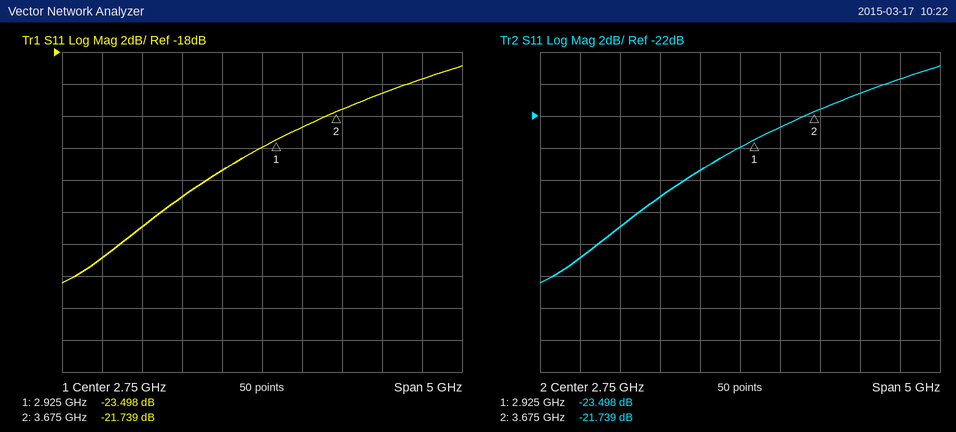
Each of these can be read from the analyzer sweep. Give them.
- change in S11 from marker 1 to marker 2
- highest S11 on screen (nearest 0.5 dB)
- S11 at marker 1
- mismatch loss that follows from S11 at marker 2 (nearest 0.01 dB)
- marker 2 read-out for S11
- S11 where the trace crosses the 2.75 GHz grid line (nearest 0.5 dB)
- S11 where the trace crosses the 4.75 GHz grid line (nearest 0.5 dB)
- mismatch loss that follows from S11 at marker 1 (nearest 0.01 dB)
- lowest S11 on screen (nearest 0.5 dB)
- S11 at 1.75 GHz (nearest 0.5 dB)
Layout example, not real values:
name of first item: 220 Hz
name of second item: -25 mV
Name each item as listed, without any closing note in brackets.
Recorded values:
change in S11 from marker 1 to marker 2: 1.759 dB
highest S11 on screen: -19.0 dB
S11 at marker 1: -23.498 dB
mismatch loss that follows from S11 at marker 2: 0.03 dB
marker 2 read-out for S11: -21.739 dB
S11 where the trace crosses the 2.75 GHz grid line: -24.0 dB
S11 where the trace crosses the 4.75 GHz grid line: -19.5 dB
mismatch loss that follows from S11 at marker 1: 0.02 dB
lowest S11 on screen: -32.5 dB
S11 at 1.75 GHz: -27.0 dB
